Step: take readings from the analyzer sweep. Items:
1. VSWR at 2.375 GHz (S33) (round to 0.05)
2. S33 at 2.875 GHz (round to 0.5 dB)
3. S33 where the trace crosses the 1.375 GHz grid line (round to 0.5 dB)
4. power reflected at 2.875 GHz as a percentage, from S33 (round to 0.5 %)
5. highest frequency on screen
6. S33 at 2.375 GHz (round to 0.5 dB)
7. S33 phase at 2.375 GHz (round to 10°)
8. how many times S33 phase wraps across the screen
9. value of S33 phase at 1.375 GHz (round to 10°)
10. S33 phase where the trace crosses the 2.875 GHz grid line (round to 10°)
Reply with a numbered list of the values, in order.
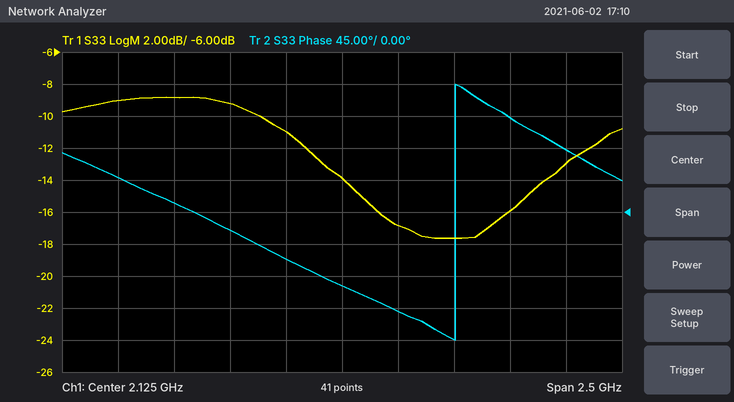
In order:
1. 1.35
2. -16.0 dB
3. -9.0 dB
4. 2.5 %
5. 3.375 GHz
6. -17.0 dB
7. -140°
8. 1
9. 10°
10. 130°
